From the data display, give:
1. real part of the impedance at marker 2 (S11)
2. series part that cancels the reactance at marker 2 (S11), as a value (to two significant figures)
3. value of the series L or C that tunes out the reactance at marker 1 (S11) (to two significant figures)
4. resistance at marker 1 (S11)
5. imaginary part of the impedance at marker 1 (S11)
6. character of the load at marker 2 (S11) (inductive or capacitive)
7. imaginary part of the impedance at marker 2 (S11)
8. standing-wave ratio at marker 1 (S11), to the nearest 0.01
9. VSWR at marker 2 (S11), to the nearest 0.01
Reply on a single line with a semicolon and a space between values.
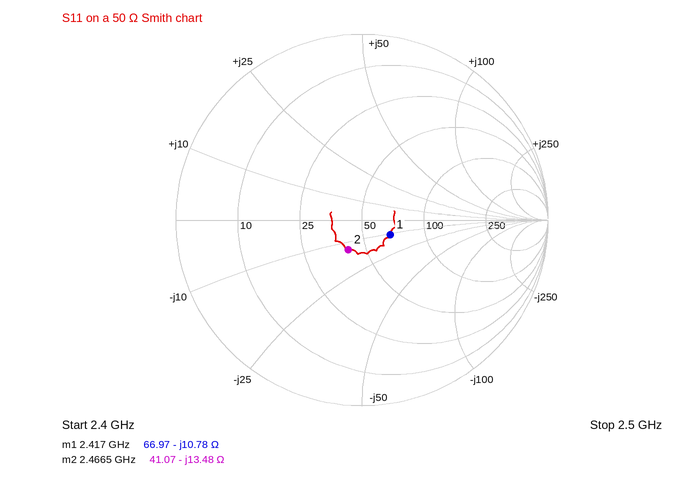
41.07 Ω; 870 pH; 710 pH; 66.97 Ω; -10.78 Ω; capacitive; -13.48 Ω; 1.41; 1.43
